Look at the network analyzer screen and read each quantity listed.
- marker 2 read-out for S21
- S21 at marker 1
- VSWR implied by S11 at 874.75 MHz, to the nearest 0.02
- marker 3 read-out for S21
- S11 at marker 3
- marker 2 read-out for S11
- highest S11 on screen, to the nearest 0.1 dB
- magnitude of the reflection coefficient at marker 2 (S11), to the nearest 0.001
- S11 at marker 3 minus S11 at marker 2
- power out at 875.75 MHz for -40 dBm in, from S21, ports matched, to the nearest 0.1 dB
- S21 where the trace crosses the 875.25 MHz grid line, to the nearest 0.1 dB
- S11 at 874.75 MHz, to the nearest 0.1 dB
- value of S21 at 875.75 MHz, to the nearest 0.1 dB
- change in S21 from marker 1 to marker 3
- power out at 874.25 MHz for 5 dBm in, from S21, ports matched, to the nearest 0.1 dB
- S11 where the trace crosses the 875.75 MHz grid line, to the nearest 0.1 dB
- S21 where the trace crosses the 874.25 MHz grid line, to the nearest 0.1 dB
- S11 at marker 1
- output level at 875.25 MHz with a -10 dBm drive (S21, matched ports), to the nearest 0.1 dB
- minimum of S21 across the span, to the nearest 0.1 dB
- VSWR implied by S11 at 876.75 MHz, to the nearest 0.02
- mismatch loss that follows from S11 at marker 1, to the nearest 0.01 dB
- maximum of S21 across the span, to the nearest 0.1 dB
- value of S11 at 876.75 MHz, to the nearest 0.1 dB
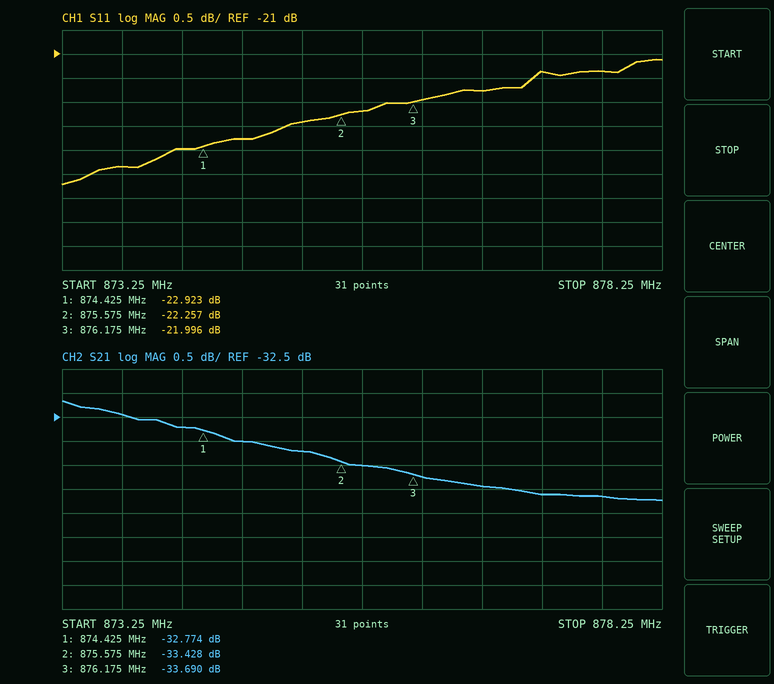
-33.428 dB
-32.774 dB
1.16
-33.690 dB
-21.996 dB
-22.257 dB
-21.1 dB
0.077
0.261 dB
-73.5 dBm
-33.2 dB
-22.8 dB
-33.5 dB
-0.916 dB
-27.7 dBm
-22.2 dB
-32.7 dB
-22.923 dB
-43.2 dBm
-34.2 dB
1.18
0.02 dB
-32.2 dB
-21.8 dB
